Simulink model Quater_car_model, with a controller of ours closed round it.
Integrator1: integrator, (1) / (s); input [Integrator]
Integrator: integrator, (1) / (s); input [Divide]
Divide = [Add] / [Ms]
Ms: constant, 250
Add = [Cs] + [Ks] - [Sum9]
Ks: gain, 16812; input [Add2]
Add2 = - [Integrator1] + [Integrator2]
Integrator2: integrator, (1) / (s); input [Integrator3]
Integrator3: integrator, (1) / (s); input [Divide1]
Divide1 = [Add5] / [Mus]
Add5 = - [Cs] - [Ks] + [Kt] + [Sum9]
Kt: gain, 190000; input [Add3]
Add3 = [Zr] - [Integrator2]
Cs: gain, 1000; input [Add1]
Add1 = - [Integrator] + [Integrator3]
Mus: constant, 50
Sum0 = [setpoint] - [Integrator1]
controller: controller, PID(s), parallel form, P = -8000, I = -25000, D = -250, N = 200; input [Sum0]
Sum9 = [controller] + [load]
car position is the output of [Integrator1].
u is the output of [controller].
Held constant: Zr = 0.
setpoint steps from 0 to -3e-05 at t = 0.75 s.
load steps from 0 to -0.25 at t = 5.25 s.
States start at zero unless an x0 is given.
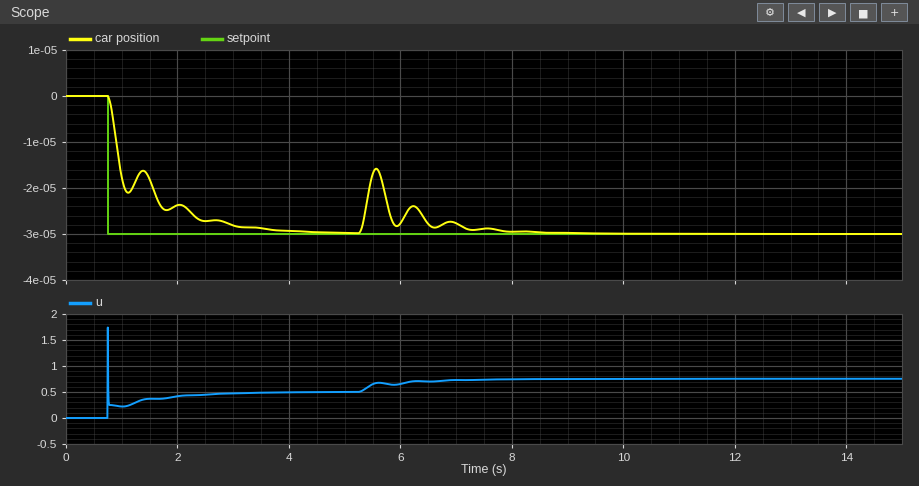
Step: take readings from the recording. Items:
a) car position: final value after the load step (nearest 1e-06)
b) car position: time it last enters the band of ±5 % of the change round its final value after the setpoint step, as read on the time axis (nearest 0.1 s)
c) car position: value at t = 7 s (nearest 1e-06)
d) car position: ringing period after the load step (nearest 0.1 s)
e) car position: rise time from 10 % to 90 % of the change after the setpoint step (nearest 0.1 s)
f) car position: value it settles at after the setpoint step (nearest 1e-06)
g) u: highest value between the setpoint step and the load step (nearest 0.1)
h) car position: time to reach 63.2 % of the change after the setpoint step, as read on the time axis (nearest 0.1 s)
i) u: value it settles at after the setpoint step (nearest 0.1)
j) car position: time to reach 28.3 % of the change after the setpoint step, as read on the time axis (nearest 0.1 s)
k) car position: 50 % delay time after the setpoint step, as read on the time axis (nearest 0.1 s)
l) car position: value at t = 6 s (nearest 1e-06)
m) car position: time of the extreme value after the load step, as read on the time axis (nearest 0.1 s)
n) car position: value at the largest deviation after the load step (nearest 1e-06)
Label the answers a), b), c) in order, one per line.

a) -0.000030
b) 3.1 s
c) -0.000028
d) 0.7 s
e) 1.6 s
f) -0.000030
g) 1.7
h) 1.0 s
i) 0.5
j) 0.9 s
k) 1.0 s
l) -0.000028
m) 5.6 s
n) -0.000016
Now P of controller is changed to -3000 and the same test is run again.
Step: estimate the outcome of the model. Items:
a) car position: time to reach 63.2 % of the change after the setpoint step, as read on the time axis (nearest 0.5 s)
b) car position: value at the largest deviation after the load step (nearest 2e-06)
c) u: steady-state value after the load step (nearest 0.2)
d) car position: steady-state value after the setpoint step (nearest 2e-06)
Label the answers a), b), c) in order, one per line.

a) 1.5 s
b) -0.000014
c) 0.8
d) -0.000030
